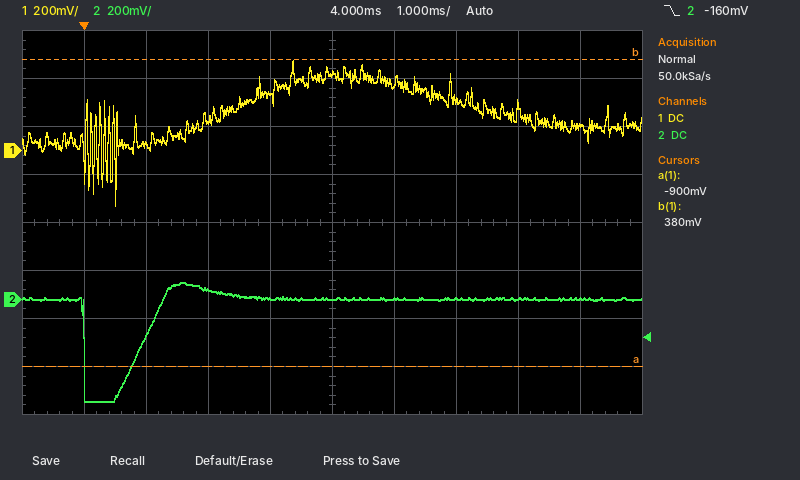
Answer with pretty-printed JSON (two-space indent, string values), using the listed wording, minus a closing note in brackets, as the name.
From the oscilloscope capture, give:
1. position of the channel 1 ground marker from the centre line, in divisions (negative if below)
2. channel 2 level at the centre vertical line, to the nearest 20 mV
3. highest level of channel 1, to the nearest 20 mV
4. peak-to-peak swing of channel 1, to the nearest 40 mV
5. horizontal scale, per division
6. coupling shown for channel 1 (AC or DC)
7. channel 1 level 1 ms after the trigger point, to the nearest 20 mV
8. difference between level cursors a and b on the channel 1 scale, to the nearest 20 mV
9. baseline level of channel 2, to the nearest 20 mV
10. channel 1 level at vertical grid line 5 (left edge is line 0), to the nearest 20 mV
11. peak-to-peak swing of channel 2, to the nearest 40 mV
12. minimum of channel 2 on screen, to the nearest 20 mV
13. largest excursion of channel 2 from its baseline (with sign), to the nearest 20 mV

{
  "position of the channel 1 ground marker from the centre line, in divisions": "+1.5 div",
  "channel 2 level at the centre vertical line, to the nearest 20 mV": "0 mV",
  "highest level of channel 1, to the nearest 20 mV": "380 mV",
  "peak-to-peak swing of channel 1, to the nearest 40 mV": "600 mV",
  "horizontal scale, per division": "1 ms",
  "coupling shown for channel 1": "DC",
  "channel 1 level 1 ms after the trigger point, to the nearest 20 mV": "20 mV",
  "difference between level cursors a and b on the channel 1 scale, to the nearest 20 mV": "1.28 V",
  "baseline level of channel 2, to the nearest 20 mV": "0 mV",
  "channel 1 level at vertical grid line 5 (left edge is line 0), to the nearest 20 mV": "320 mV",
  "peak-to-peak swing of channel 2, to the nearest 40 mV": "480 mV",
  "minimum of channel 2 on screen, to the nearest 20 mV": "-420 mV",
  "largest excursion of channel 2 from its baseline (with sign), to the nearest 20 mV": "-420 mV"
}
